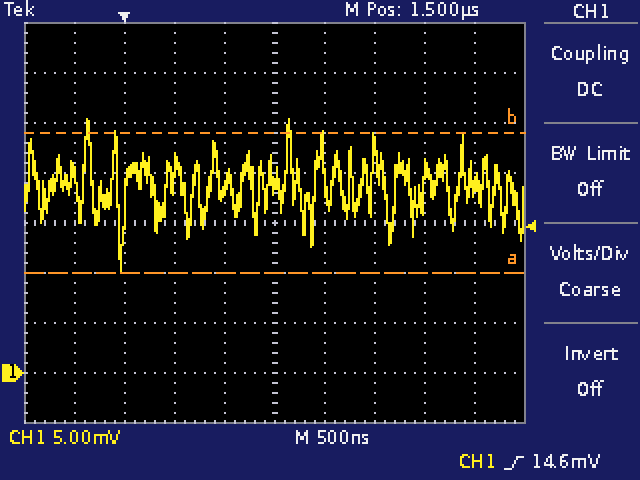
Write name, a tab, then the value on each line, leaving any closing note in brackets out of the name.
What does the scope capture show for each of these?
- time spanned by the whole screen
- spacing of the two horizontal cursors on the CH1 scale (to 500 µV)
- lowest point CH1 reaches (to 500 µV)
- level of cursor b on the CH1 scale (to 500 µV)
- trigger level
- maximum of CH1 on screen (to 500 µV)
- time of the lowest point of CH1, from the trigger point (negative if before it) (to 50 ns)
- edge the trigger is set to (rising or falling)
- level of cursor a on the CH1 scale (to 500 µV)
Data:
time spanned by the whole screen	5 µs
spacing of the two horizontal cursors on the CH1 scale	14.0 mV
lowest point CH1 reaches	10.0 mV
level of cursor b on the CH1 scale	24.0 mV
trigger level	14.6 mV
maximum of CH1 on screen	25.5 mV
time of the lowest point of CH1, from the trigger point (negative if before it)	-50 ns
edge the trigger is set to	rising
level of cursor a on the CH1 scale	10.0 mV
